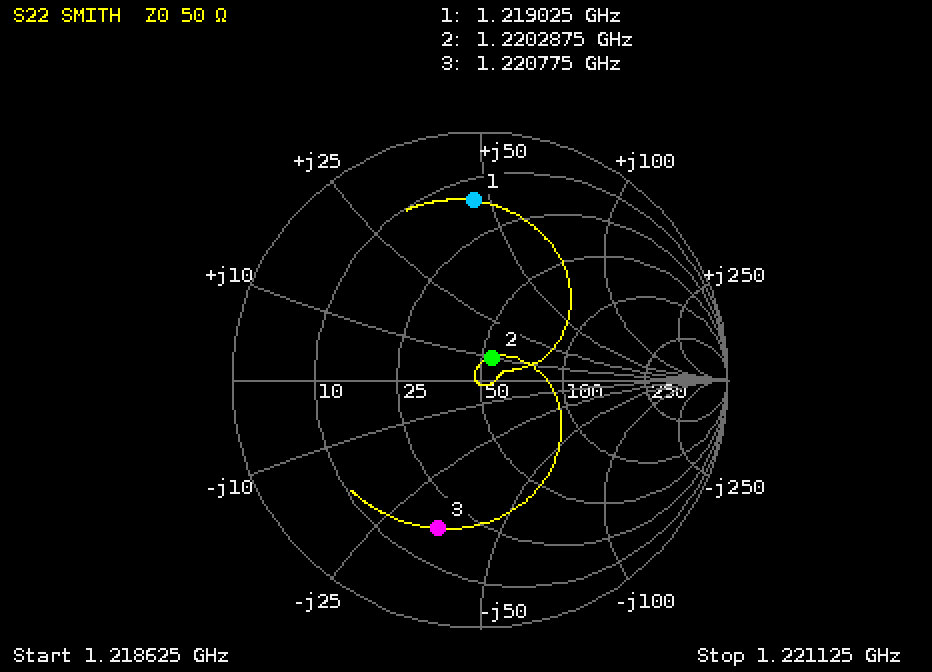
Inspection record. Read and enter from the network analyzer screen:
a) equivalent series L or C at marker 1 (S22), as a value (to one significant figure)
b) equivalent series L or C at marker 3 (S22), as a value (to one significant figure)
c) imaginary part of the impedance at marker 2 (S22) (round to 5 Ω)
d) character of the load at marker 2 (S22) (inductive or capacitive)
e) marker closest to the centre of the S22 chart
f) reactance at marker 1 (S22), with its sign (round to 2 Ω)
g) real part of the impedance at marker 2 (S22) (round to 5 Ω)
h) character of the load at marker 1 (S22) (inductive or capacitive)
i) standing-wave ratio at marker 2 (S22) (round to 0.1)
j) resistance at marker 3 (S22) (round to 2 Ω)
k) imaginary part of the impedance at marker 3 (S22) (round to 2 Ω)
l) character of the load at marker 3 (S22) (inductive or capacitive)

6 nH
4 pF
+10 Ω
inductive
marker 2
+46 Ω
55 Ω
inductive
1.2
18 Ω
-34 Ω
capacitive
